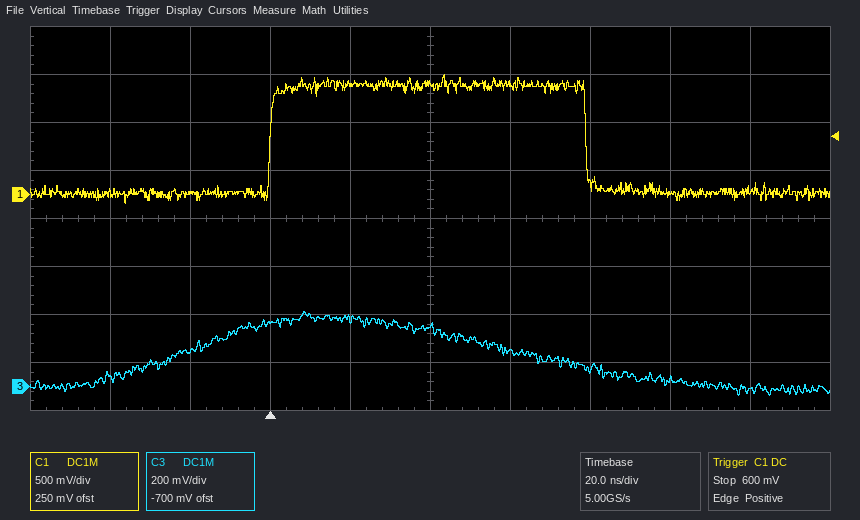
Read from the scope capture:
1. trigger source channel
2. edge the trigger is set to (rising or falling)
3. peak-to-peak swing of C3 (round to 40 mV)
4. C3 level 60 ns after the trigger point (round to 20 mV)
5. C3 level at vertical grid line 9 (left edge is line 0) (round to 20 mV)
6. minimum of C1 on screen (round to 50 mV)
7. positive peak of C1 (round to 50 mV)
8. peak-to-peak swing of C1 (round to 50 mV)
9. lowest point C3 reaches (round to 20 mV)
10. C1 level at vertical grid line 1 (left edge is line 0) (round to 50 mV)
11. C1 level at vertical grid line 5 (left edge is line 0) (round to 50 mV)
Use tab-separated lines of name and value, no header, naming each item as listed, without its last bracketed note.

trigger source channel	C1
edge the trigger is set to	rising
peak-to-peak swing of C3	360 mV
C3 level 60 ns after the trigger point	140 mV
C3 level at vertical grid line 9 (left edge is line 0)	-20 mV
minimum of C1 on screen	-100 mV
positive peak of C1	1.25 V
peak-to-peak swing of C1	1.35 V
lowest point C3 reaches	-40 mV
C1 level at vertical grid line 1 (left edge is line 0)	0 mV
C1 level at vertical grid line 5 (left edge is line 0)	1.15 V
